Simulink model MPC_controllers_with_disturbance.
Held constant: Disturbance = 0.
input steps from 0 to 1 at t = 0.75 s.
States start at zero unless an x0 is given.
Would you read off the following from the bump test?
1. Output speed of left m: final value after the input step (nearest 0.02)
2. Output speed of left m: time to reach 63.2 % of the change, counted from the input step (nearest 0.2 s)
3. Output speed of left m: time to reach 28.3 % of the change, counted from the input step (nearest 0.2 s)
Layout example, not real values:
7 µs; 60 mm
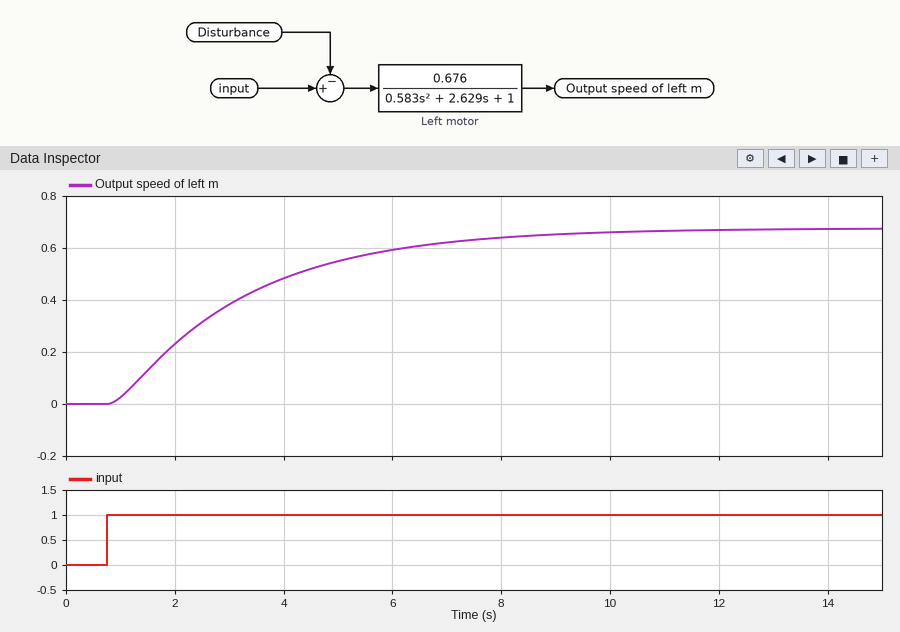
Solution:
0.68; 2.6 s; 1.0 s
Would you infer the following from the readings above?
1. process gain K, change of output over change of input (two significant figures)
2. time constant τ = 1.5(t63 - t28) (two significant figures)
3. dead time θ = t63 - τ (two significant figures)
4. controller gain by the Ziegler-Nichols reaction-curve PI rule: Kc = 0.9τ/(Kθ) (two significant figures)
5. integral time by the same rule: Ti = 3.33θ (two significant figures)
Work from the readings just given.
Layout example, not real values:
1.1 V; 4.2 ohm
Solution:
0.68; 2.4 s; 0.20 s; 16; 0.67 s
